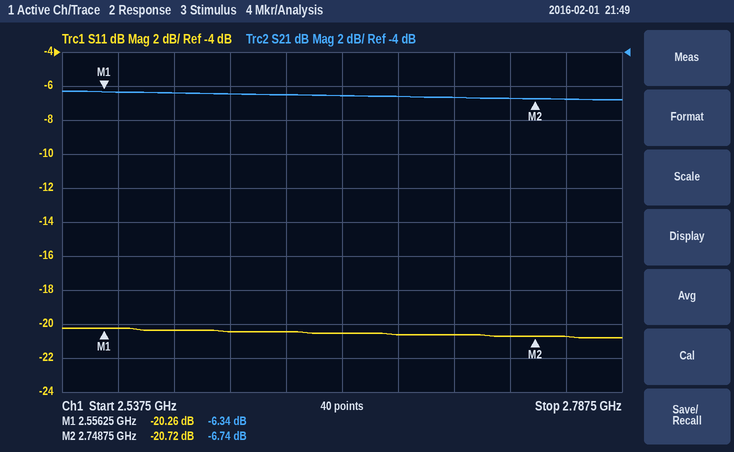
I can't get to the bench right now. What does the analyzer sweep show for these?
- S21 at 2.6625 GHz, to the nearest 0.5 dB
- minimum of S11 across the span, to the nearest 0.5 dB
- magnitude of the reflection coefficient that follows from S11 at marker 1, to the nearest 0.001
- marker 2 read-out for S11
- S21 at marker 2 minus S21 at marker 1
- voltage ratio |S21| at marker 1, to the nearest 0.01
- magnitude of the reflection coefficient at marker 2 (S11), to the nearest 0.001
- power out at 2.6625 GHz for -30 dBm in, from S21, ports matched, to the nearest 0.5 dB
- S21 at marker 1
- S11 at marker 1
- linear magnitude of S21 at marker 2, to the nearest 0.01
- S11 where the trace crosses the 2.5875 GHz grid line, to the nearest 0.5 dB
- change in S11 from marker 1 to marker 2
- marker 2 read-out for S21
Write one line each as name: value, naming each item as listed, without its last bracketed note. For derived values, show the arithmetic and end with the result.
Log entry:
S21 at 2.6625 GHz, to the nearest 0.5 dB: -6.5 dB
minimum of S11 across the span, to the nearest 0.5 dB: -21.0 dB
magnitude of the reflection coefficient that follows from S11 at marker 1, to the nearest 0.001: 10^(-20.26/20) ≈ 0.097
marker 2 read-out for S11: -20.72 dB
S21 at marker 2 minus S21 at marker 1: -6.74 − (-6.34) = -0.40 dB
voltage ratio |S21| at marker 1, to the nearest 0.01: 10^(-6.34/20) ≈ 0.48
magnitude of the reflection coefficient at marker 2 (S11), to the nearest 0.001: 10^(-20.72/20) ≈ 0.092
power out at 2.6625 GHz for -30 dBm in, from S21, ports matched, to the nearest 0.5 dB: -30 dBm + (-6.5 dB) = -36.5 dBm
S21 at marker 1: -6.34 dB
S11 at marker 1: -20.26 dB
linear magnitude of S21 at marker 2, to the nearest 0.01: 10^(-6.74/20) ≈ 0.46
S11 where the trace crosses the 2.5875 GHz grid line, to the nearest 0.5 dB: -20.5 dB
change in S11 from marker 1 to marker 2: -20.72 − (-20.26) = -0.46 dB
marker 2 read-out for S21: -6.74 dB
